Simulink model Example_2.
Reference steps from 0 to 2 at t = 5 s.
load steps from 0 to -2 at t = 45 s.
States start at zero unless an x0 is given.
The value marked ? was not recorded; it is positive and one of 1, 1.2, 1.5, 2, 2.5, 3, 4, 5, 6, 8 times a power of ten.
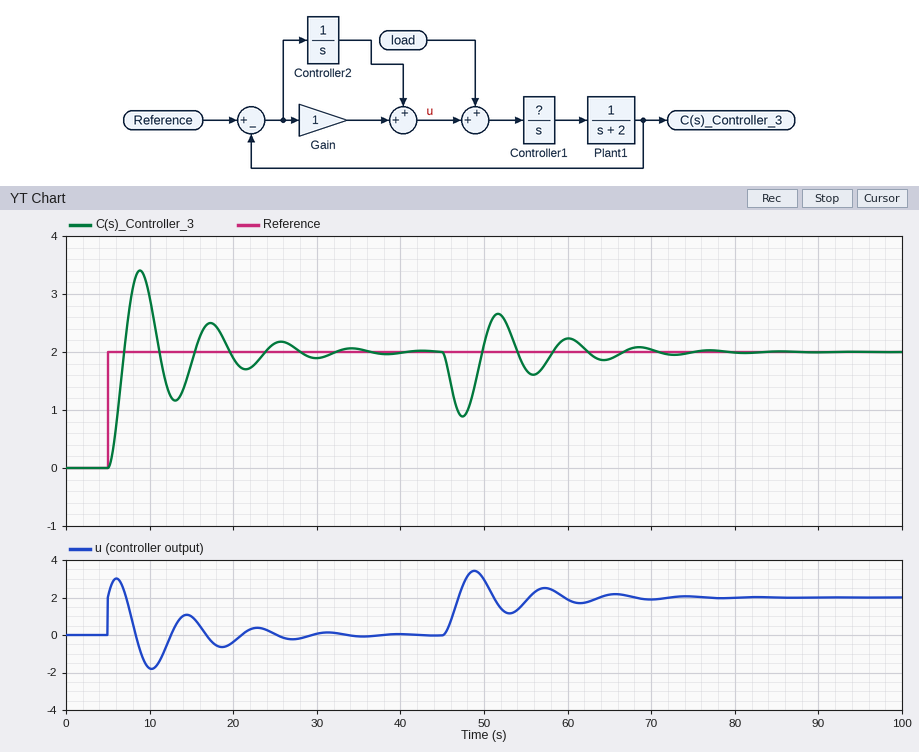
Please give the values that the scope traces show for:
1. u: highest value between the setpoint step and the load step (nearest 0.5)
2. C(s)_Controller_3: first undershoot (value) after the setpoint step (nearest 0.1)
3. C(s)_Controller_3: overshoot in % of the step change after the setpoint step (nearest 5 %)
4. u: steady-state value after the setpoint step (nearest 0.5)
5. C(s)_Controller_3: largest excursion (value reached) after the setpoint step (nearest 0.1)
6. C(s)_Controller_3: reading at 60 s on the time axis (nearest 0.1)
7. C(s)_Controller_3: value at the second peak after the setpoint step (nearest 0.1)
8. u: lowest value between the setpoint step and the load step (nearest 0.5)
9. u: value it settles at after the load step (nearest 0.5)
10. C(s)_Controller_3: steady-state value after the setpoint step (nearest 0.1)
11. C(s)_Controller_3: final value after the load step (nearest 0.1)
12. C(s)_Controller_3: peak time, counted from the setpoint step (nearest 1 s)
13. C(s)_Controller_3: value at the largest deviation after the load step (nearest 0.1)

3.0
1.2
70 %
0.0
3.4
2.2
2.5
-2.0
2.0
2.0
2.0
4 s
0.9
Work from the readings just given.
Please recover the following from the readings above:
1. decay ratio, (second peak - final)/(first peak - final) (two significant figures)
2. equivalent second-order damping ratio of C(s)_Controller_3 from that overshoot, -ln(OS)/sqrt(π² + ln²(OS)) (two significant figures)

0.36
0.11
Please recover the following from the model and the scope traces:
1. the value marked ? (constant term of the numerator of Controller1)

1
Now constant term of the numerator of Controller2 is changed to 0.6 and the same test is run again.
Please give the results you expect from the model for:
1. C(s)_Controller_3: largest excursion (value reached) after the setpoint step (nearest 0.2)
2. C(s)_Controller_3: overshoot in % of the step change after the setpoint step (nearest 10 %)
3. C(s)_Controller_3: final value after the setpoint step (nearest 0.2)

3.0
50 %
2.0
